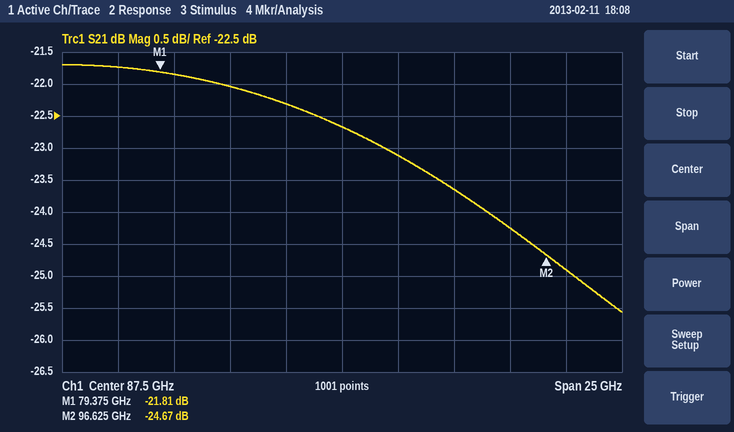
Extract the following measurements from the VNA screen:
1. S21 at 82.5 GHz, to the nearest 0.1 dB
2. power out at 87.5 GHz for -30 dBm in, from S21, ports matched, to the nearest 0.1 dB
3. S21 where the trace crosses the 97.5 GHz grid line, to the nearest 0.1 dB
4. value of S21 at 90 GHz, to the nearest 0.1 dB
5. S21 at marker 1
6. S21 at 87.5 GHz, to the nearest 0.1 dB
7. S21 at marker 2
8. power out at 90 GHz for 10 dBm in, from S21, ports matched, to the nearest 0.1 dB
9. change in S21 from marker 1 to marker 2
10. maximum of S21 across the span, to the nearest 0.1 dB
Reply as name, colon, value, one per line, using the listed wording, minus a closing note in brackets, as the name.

S21 at 82.5 GHz, to the nearest 0.1 dB: -22.0 dB
power out at 87.5 GHz for -30 dBm in, from S21, ports matched, to the nearest 0.1 dB: -52.7 dBm
S21 where the trace crosses the 97.5 GHz grid line, to the nearest 0.1 dB: -24.9 dB
value of S21 at 90 GHz, to the nearest 0.1 dB: -23.1 dB
S21 at marker 1: -21.81 dB
S21 at 87.5 GHz, to the nearest 0.1 dB: -22.7 dB
S21 at marker 2: -24.67 dB
power out at 90 GHz for 10 dBm in, from S21, ports matched, to the nearest 0.1 dB: -13.1 dBm
change in S21 from marker 1 to marker 2: -2.86 dB
maximum of S21 across the span, to the nearest 0.1 dB: -21.7 dB
